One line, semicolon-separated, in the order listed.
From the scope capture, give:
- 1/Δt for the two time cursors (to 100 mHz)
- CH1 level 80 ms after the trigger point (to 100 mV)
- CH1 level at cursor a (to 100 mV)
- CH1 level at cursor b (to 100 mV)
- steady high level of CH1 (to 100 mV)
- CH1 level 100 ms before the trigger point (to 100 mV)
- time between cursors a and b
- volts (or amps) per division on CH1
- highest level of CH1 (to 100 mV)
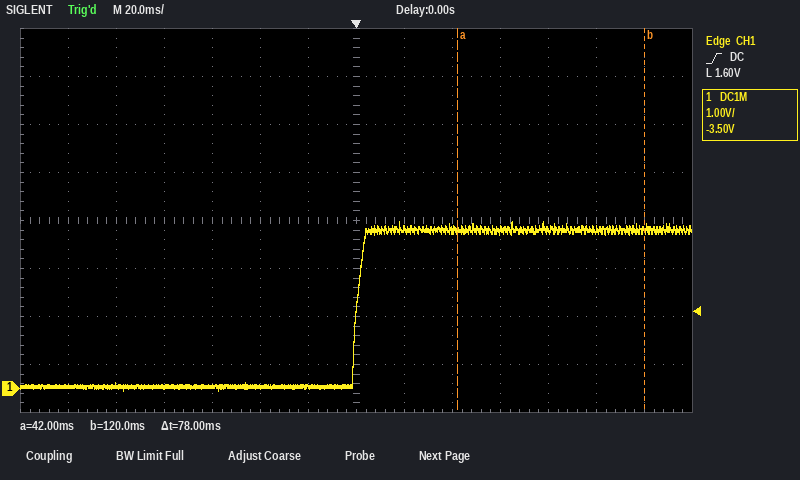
12.8 Hz; 3.3 V; 3.3 V; 3.3 V; 3.3 V; 100 mV; 78 ms; 1 V; 3.5 V
